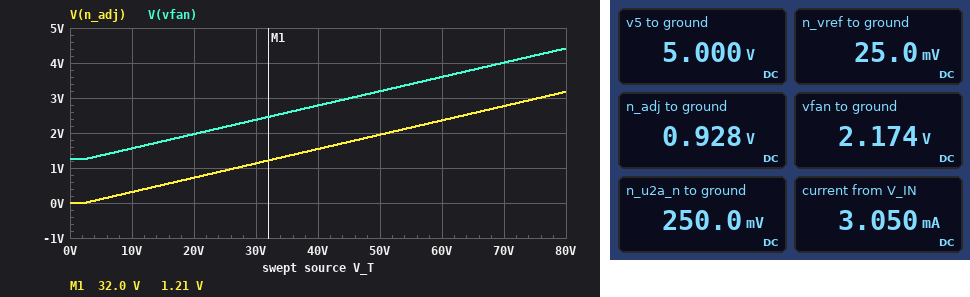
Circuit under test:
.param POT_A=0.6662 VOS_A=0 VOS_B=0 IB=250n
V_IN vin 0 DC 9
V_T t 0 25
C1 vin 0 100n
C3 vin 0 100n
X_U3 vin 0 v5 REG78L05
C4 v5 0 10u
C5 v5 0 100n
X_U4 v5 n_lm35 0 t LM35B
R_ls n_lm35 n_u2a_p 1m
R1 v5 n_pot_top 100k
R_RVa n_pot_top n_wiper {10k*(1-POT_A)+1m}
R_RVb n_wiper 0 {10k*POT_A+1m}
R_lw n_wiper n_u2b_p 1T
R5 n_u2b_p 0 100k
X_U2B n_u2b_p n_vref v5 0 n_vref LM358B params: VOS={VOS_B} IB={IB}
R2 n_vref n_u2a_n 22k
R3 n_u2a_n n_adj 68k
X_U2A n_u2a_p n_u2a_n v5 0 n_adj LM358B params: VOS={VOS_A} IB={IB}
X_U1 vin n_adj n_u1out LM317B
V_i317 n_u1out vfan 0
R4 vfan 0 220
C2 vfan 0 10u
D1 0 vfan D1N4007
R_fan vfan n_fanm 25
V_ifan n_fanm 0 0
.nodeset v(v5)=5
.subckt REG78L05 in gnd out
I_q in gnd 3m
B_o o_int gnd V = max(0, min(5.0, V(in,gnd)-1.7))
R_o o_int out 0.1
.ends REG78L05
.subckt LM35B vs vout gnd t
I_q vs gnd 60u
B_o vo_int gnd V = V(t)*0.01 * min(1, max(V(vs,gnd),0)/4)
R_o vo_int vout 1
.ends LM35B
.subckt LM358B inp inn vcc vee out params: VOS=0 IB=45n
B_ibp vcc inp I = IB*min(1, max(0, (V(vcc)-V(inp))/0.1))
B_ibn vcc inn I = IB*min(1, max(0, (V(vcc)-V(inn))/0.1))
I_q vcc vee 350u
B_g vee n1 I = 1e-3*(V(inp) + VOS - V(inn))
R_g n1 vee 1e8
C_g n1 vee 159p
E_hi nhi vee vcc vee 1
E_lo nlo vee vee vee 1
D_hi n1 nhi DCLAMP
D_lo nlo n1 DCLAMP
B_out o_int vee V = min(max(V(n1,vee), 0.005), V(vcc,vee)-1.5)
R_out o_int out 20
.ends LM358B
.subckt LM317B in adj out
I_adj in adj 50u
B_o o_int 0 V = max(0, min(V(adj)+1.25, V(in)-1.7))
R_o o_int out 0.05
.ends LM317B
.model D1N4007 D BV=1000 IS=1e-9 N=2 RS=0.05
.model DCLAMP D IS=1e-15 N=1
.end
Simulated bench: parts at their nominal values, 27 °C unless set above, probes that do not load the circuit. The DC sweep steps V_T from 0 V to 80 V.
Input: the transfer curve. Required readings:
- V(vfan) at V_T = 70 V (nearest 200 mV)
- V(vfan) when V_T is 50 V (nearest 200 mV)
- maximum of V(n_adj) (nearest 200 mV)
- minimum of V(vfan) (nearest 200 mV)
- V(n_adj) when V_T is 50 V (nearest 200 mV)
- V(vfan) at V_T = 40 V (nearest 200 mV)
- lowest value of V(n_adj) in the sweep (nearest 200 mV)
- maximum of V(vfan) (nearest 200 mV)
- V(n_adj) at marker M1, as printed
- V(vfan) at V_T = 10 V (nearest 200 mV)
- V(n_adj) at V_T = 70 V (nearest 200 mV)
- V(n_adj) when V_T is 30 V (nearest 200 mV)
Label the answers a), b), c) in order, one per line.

a) 4.0 V
b) 3.2 V
c) 3.2 V
d) 1.2 V
e) 2.0 V
f) 2.8 V
g) 0 V
h) 4.4 V
i) 1.21 V
j) 1.6 V
k) 2.8 V
l) 1.2 V
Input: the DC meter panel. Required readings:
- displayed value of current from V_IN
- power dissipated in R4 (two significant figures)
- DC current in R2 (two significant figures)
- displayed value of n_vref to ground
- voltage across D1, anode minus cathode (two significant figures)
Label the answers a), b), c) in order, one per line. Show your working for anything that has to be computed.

a) 3.050 mA
b) (2.174 V)^2 / 220 Ω = 21 mW
c) (250 mV - 25 mV) / 22 kΩ = 10 µA
d) 25.0 mV
e) 0 V - 2.174 V = -2.2 V
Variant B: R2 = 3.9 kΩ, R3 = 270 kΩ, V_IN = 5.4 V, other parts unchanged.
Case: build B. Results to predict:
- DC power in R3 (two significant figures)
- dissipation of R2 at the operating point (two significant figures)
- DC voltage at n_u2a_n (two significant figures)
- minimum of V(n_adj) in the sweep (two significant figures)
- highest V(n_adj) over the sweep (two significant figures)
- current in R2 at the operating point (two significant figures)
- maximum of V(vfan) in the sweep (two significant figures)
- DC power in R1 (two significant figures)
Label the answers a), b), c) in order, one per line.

a) 17 µW
b) 260 nW
c) 57 mV
d) 6.0 mV
e) 2.2 V
f) 8.2 µA
g) 3.4 V
h) 110 µW
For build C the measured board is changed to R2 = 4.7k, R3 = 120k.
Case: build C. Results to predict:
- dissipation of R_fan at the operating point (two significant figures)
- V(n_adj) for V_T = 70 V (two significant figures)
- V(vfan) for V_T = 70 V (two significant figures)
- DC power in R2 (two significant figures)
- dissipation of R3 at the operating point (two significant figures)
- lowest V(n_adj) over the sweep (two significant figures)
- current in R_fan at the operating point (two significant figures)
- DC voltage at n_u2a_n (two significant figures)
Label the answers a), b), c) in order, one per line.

a) 900 mW
b) 3.5 V
c) 4.7 V
d) 3.7 µW
e) 93 µW
f) 6.0 mV
g) 190 mA
h) 160 mV
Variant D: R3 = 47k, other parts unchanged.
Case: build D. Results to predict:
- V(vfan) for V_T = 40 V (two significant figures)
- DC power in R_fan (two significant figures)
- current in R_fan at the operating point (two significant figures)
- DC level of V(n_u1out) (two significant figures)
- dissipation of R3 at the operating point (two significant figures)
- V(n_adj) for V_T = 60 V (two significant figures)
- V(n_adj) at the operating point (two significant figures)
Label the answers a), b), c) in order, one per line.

a) 2.4 V
b) 150 mW
c) 79 mA
d) 2.0 V
e) 4.7 µW
f) 1.8 V
g) 720 mV
